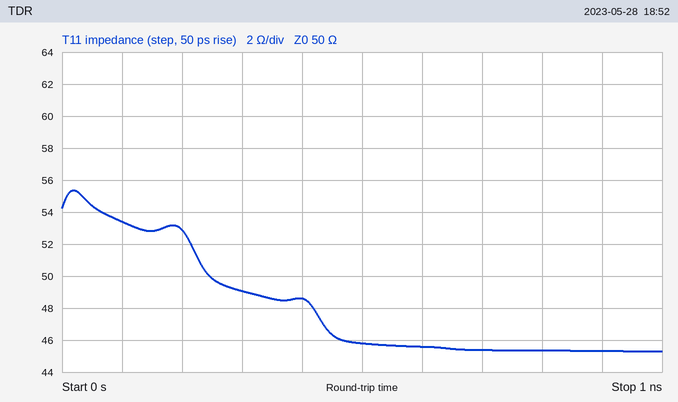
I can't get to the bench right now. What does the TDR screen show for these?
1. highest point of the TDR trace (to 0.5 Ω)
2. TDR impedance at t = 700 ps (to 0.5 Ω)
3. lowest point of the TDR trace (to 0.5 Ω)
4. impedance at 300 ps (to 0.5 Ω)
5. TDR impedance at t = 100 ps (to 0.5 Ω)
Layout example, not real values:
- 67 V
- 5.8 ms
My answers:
- 55.5 Ω
- 45.5 Ω
- 45.5 Ω
- 49.0 Ω
- 53.5 Ω
